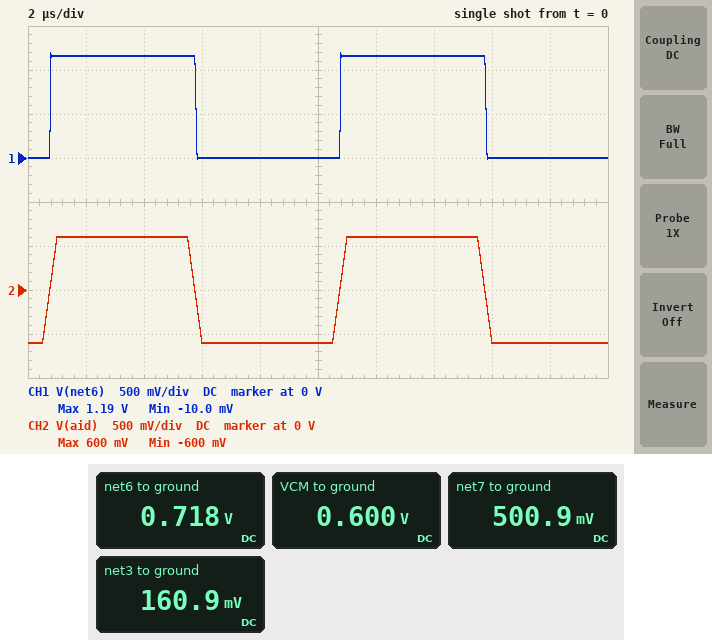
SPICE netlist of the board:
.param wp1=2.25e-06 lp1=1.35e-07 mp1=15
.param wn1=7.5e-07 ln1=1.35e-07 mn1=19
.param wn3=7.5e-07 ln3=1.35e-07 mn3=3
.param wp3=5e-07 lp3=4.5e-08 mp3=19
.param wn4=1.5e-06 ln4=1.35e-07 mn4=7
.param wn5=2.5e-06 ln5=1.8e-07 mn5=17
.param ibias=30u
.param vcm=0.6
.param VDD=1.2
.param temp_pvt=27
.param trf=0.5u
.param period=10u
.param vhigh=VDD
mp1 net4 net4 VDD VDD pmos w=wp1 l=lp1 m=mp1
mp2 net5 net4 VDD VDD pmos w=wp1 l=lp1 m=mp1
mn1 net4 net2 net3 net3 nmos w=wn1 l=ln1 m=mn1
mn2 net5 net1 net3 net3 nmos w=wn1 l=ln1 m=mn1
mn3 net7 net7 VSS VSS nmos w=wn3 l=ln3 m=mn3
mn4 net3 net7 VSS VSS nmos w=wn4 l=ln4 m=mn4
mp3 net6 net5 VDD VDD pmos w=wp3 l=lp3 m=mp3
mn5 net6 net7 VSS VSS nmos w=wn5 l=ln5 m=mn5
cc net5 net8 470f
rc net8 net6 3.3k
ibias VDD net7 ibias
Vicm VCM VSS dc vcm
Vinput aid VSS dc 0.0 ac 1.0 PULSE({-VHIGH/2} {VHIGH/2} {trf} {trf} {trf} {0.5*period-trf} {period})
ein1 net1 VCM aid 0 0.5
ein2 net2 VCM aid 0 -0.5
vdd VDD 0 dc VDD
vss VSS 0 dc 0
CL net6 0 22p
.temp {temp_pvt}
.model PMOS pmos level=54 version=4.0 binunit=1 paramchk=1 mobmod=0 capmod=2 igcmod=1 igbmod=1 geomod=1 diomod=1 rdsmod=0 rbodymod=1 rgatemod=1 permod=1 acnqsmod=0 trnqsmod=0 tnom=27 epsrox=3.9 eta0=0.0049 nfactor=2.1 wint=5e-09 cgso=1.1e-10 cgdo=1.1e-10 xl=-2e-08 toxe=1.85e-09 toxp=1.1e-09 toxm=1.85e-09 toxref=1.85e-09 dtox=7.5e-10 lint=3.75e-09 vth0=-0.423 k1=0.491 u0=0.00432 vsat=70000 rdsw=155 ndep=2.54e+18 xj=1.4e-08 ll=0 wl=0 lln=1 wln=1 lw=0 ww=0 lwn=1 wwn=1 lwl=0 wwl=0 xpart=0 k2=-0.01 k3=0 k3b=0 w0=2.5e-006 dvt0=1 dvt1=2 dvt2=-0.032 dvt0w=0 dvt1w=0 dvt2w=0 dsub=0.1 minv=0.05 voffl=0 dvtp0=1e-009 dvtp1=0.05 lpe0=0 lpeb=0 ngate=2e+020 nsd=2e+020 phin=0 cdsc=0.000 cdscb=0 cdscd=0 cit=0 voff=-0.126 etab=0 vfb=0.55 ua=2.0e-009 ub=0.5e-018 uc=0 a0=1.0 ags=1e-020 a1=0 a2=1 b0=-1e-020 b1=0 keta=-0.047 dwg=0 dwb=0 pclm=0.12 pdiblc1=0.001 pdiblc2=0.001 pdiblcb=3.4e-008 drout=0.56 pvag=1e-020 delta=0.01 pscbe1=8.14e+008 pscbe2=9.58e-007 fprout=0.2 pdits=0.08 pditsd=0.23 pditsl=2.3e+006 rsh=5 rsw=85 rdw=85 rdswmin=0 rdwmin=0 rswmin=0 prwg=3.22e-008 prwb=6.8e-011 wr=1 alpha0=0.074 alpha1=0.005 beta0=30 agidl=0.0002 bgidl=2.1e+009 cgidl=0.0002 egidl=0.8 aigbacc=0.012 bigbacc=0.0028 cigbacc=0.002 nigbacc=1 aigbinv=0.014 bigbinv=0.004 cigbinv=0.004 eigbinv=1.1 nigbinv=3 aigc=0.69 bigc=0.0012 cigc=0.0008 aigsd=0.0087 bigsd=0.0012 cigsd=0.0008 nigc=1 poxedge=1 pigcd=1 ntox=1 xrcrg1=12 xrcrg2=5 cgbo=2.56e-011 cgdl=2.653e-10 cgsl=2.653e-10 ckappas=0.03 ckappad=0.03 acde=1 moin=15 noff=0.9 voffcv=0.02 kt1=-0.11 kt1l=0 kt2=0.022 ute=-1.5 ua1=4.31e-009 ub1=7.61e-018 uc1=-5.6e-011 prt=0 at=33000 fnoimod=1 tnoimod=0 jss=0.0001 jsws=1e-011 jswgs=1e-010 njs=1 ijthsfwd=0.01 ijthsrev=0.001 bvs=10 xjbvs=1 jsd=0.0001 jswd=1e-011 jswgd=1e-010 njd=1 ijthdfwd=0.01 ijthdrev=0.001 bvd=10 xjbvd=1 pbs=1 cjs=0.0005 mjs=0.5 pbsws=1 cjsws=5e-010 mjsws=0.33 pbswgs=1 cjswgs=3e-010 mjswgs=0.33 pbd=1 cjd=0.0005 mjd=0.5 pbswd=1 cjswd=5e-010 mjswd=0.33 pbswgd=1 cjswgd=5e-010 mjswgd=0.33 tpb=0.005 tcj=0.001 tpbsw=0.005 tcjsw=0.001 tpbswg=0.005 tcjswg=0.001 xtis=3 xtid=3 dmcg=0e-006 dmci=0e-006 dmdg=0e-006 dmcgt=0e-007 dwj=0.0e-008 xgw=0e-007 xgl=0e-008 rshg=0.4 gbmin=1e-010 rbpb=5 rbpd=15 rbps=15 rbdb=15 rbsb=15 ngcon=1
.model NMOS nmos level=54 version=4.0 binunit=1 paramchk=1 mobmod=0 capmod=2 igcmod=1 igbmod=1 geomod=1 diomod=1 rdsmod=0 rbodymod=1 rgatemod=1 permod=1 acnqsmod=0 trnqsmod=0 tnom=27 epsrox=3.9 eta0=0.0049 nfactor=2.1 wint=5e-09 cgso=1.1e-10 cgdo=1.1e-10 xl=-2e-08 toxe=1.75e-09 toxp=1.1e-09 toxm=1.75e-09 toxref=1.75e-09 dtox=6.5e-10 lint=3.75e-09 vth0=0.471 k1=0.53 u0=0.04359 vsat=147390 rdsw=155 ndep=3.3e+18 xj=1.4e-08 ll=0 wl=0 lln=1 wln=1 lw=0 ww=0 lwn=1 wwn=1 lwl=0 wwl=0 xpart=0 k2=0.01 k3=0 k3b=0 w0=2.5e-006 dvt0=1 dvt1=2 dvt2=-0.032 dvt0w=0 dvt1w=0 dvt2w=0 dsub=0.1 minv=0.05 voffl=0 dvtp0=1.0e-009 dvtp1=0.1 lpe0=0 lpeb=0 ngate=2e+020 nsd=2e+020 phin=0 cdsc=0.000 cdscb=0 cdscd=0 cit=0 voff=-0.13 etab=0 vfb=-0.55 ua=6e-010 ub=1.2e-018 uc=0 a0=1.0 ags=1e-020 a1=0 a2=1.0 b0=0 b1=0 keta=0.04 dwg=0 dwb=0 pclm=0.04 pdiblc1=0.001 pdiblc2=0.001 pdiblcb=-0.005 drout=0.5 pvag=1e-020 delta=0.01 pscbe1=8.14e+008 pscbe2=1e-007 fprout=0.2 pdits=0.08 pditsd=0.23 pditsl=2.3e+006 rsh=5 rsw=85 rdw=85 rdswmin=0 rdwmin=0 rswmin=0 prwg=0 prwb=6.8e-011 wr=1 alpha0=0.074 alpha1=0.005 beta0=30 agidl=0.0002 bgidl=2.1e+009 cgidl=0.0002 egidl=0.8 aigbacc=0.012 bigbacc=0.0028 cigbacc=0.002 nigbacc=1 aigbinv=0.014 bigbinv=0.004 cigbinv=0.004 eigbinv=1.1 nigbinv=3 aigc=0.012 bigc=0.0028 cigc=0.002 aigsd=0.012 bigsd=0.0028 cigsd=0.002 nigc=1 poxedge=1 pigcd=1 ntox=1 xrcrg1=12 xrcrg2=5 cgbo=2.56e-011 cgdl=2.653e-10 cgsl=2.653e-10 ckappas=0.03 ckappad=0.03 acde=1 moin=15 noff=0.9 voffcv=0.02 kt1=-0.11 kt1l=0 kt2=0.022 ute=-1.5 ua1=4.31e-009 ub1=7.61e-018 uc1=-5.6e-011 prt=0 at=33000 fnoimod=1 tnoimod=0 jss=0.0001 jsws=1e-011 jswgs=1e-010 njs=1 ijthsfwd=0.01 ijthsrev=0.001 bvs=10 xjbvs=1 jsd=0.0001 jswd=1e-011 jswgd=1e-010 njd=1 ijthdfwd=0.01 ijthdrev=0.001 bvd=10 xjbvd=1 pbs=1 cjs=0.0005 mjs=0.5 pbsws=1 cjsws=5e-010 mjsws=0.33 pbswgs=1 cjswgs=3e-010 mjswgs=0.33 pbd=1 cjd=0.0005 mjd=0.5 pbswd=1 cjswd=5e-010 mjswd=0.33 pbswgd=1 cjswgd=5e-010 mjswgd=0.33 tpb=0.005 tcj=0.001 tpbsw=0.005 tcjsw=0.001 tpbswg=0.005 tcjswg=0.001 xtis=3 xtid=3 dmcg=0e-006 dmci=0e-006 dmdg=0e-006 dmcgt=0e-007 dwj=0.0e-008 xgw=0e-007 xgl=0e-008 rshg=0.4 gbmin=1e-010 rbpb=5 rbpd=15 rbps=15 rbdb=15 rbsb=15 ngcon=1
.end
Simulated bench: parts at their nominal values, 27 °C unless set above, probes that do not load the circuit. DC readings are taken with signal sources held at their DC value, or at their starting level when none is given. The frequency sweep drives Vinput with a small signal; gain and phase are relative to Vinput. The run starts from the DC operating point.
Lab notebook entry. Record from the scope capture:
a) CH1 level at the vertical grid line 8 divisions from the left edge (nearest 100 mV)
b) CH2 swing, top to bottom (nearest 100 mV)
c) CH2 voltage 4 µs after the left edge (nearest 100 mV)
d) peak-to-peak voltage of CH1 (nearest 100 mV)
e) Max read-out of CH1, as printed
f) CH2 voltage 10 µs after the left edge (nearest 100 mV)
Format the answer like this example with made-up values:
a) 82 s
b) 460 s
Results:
a) 0 V
b) 1.2 V
c) 600 mV
d) 1.2 V
e) 1.19 V
f) -600 mV
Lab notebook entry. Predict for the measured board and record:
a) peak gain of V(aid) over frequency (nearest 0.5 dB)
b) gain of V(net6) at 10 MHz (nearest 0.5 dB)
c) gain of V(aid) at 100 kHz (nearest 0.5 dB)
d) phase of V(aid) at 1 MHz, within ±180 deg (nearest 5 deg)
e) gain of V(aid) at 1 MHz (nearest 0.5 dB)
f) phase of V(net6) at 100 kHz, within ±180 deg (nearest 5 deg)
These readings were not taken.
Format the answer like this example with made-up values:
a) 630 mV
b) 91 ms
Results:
a) 0 dB
b) 28.5 dB
c) 0 dB
d) 0 deg
e) 0 dB
f) -5 deg
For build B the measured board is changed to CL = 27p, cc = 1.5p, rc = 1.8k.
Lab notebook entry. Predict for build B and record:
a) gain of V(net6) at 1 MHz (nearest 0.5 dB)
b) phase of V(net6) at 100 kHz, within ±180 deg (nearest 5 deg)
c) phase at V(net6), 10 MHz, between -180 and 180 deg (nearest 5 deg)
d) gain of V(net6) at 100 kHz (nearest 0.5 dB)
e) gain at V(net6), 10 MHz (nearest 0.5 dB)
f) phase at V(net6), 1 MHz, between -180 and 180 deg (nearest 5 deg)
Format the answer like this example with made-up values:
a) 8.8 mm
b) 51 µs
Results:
a) 39.0 dB
b) -15 deg
c) -100 deg
d) 48.0 dB
e) 19.0 dB
f) -70 deg
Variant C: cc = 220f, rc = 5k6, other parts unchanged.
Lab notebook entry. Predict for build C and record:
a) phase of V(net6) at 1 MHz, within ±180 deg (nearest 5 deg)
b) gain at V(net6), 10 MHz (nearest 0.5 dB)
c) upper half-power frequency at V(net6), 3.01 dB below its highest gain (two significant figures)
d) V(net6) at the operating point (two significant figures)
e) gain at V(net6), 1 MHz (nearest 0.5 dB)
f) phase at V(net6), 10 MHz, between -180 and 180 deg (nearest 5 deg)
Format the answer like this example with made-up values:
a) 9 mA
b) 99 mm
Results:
a) -30 deg
b) 33.5 dB
c) 1.9 MHz
d) 720 mV
e) 47.5 dB
f) -90 deg
